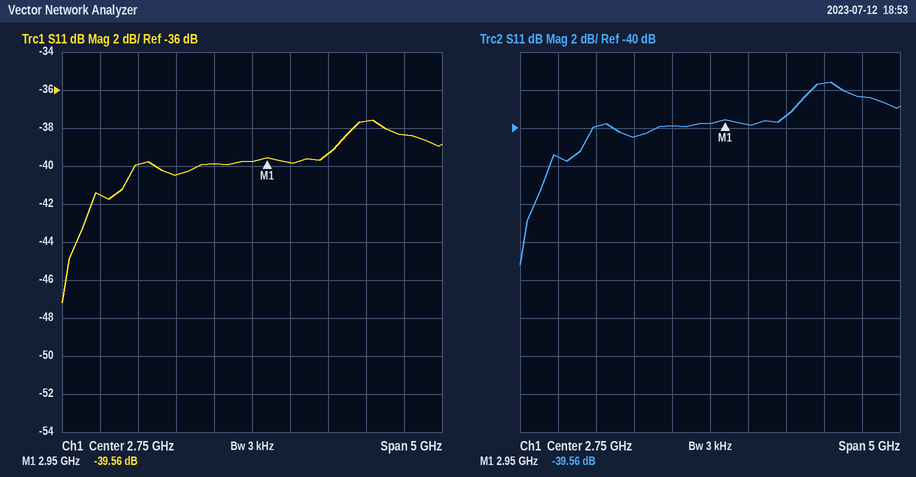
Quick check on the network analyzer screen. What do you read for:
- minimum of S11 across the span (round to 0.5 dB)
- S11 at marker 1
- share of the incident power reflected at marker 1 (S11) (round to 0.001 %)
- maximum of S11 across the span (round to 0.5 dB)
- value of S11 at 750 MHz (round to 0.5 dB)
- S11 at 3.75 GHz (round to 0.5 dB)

-47.0 dB
-39.56 dB
0.011 %
-37.5 dB
-41.5 dB
-39.5 dB
